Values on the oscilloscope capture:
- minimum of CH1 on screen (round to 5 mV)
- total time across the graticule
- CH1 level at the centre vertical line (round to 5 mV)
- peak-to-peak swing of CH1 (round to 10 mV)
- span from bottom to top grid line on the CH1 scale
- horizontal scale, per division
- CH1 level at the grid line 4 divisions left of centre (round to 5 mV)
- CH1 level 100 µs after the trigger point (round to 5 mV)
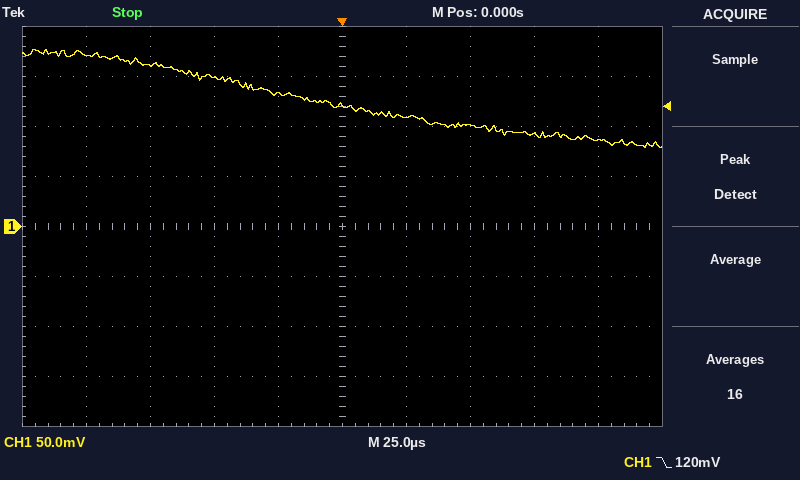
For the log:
80 mV
250 µs
120 mV
100 mV
400 mV
25 µs
170 mV
85 mV
